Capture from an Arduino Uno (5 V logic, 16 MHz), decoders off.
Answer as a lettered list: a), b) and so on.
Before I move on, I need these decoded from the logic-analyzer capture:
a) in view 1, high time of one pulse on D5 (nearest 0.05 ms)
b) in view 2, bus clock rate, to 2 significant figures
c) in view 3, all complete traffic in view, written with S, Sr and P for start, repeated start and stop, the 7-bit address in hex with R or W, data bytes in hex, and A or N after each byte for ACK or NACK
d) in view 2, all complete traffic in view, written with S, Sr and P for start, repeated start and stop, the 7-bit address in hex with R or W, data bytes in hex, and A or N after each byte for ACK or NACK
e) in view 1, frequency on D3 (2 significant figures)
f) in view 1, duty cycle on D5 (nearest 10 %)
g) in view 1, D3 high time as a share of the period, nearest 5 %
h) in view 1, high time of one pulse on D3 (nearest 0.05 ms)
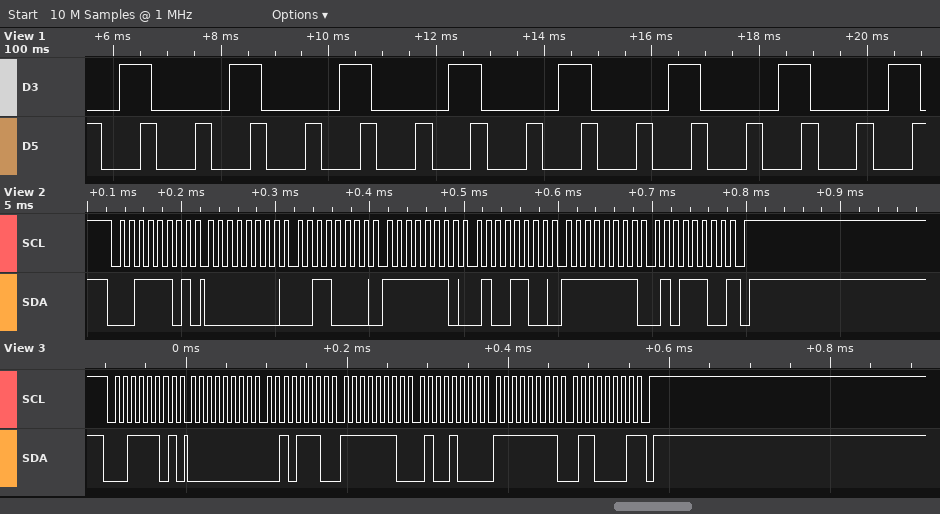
a) 0.30 ms
b) 100 kHz
c) S 1ER A 00 A 2E A FE A 48 A FF A 61 N P
d) S 1ER A 00 A 30 A FE A 4C A FF A 5C N P
e) 490 Hz
f) 30 %
g) 30 %
h) 0.60 ms
